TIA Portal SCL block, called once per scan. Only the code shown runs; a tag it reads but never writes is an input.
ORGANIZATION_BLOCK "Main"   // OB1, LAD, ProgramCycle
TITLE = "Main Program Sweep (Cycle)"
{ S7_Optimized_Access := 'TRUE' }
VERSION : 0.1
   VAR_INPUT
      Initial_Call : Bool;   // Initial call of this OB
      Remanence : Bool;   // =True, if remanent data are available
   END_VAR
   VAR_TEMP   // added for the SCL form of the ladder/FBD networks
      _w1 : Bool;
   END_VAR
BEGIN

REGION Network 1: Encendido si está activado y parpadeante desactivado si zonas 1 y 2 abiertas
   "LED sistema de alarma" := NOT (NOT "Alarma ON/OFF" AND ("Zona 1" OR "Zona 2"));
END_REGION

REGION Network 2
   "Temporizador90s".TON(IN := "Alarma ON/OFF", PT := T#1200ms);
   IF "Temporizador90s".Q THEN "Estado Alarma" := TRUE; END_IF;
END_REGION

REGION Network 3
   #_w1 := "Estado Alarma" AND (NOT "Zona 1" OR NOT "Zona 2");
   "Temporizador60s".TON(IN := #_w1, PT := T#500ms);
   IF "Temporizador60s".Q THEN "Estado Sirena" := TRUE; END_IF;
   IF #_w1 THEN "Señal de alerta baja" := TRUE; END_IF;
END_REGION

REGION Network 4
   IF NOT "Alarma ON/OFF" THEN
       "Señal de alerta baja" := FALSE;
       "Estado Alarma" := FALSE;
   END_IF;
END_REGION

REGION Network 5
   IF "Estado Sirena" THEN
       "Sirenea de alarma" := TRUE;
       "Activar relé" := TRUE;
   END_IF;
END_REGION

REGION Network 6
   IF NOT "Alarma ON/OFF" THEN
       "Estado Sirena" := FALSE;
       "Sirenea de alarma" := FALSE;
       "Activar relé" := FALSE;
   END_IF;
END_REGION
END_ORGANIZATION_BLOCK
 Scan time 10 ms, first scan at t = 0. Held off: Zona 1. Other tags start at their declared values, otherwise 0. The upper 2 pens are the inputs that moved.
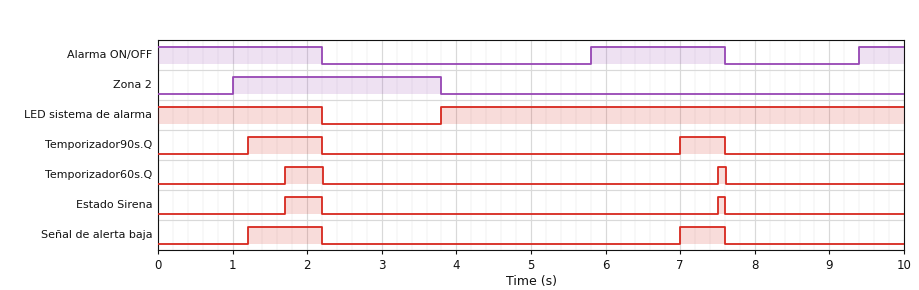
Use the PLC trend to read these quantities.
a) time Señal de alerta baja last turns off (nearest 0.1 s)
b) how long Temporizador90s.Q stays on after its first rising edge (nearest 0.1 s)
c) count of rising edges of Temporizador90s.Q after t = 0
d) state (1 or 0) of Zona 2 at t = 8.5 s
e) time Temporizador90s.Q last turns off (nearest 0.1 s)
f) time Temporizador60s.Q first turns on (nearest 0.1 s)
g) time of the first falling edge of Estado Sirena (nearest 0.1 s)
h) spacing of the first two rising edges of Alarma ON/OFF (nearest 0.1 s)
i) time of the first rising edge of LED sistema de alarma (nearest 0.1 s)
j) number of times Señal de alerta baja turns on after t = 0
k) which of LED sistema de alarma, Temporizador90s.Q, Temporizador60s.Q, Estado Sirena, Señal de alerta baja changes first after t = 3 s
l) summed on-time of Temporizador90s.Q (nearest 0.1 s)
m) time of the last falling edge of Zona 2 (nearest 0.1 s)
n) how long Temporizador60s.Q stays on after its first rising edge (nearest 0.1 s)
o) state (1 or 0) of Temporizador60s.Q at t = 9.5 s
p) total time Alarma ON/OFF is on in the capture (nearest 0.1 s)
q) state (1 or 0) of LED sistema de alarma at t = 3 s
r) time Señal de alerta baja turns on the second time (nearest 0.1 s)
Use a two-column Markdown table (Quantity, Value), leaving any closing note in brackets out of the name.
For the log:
| Quantity | Value |
|---|---|
| time Señal de alerta baja last turns off | 7.6 s |
| how long Temporizador90s.Q stays on after its first rising edge | 1.0 s |
| count of rising edges of Temporizador90s.Q after t = 0 | 2 |
| state (1 or 0) of Zona 2 at t = 8.5 s | 0 |
| time Temporizador90s.Q last turns off | 7.6 s |
| time Temporizador60s.Q first turns on | 1.7 s |
| time of the first falling edge of Estado Sirena | 2.2 s |
| spacing of the first two rising edges of Alarma ON/OFF | 3.6 s |
| time of the first rising edge of LED sistema de alarma | 3.8 s |
| number of times Señal de alerta baja turns on after t = 0 | 2 |
| which of LED sistema de alarma, Temporizador90s.Q, Temporizador60s.Q, Estado Sirena, Señal de alerta baja changes first after t = 3 s | LED sistema de alarma |
| summed on-time of Temporizador90s.Q | 1.6 s |
| time of the last falling edge of Zona 2 | 3.8 s |
| how long Temporizador60s.Q stays on after its first rising edge | 0.5 s |
| state (1 or 0) of Temporizador60s.Q at t = 9.5 s | 0 |
| total time Alarma ON/OFF is on in the capture | 4.6 s |
| state (1 or 0) of LED sistema de alarma at t = 3 s | 0 |
| time Señal de alerta baja turns on the second time | 7.0 s |
